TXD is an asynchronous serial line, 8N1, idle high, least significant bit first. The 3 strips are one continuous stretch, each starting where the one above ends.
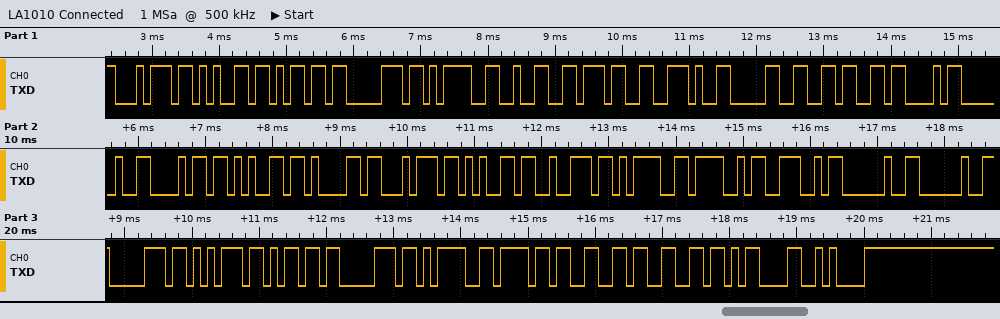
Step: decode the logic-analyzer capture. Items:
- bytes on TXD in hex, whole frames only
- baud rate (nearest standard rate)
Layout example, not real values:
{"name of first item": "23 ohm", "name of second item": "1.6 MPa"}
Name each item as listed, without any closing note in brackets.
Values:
{"bytes on TXD in hex, whole frames only": "74 65 6D 70 3D 32 37 2E 30 36 43 20 68 65 61 74 65 72 3D 4F 4E 20 20 70 75 6D 70 3D 6F 66 66 0D 0A", "baud rate": "9600 baud"}
